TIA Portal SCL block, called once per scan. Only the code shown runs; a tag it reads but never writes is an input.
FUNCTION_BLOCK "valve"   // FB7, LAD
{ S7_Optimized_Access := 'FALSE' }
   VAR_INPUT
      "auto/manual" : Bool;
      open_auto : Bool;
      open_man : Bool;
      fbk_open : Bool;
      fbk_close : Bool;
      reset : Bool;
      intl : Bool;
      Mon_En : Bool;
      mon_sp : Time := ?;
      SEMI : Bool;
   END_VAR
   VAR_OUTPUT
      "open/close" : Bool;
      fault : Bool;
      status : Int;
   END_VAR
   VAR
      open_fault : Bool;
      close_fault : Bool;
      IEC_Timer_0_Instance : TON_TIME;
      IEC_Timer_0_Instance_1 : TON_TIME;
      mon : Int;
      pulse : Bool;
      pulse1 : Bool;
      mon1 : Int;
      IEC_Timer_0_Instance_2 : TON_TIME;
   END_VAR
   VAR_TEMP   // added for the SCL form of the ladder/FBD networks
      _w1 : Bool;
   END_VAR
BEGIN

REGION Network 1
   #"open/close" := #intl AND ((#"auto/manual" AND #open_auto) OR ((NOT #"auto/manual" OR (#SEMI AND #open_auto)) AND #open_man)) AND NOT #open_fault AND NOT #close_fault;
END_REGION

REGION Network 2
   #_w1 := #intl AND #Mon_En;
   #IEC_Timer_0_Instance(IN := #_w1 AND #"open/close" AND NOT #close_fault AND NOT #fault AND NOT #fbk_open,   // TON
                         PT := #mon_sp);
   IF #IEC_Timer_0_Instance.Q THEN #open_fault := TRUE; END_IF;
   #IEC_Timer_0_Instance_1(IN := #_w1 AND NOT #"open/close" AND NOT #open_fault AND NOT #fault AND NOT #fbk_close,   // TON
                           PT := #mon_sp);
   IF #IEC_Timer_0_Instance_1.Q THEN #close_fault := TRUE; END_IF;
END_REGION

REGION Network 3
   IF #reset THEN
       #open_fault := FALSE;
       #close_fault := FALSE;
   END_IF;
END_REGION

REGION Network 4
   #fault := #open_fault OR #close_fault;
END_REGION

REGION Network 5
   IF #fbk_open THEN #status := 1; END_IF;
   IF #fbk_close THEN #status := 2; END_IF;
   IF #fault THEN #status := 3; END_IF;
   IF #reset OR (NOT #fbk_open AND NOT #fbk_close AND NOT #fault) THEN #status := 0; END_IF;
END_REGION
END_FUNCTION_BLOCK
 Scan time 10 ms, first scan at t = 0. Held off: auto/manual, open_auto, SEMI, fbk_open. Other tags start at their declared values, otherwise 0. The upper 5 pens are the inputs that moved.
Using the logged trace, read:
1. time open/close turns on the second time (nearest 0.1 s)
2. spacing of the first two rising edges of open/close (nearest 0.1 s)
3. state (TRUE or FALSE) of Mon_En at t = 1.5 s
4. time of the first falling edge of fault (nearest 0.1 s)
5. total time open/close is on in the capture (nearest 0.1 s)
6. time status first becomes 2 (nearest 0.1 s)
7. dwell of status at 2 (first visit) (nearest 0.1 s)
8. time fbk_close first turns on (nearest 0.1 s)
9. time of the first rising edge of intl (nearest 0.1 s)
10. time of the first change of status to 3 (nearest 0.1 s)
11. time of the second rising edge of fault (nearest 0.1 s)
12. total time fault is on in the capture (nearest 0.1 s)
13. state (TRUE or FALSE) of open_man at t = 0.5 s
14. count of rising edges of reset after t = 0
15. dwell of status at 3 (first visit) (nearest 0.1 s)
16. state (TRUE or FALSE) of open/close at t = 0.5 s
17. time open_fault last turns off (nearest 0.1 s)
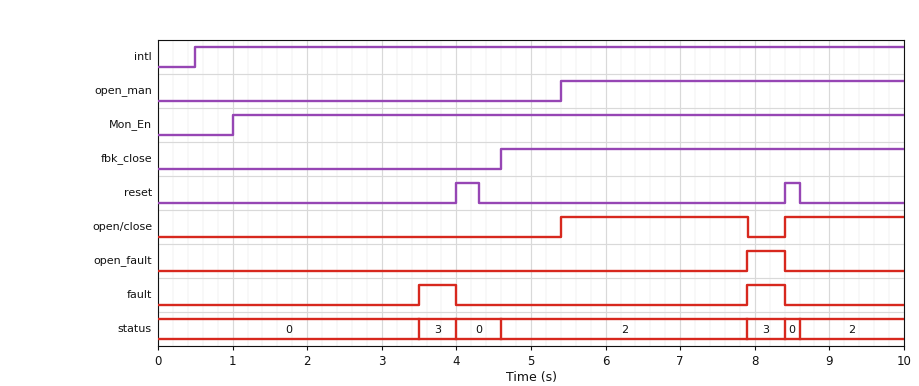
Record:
8.4 s
3.0 s
TRUE
4.0 s
4.1 s
4.6 s
3.3 s
4.6 s
0.5 s
3.5 s
7.9 s
1.0 s
FALSE
2
0.5 s
FALSE
8.4 s
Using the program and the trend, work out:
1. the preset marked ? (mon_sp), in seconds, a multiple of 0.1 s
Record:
2.5 s
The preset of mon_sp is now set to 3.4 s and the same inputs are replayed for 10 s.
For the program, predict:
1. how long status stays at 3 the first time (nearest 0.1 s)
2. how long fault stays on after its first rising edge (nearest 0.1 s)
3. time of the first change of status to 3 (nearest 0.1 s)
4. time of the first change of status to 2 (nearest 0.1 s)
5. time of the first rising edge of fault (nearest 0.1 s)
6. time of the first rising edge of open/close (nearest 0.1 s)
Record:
4.0 s
4.0 s
4.4 s
8.6 s
4.4 s
8.4 s
